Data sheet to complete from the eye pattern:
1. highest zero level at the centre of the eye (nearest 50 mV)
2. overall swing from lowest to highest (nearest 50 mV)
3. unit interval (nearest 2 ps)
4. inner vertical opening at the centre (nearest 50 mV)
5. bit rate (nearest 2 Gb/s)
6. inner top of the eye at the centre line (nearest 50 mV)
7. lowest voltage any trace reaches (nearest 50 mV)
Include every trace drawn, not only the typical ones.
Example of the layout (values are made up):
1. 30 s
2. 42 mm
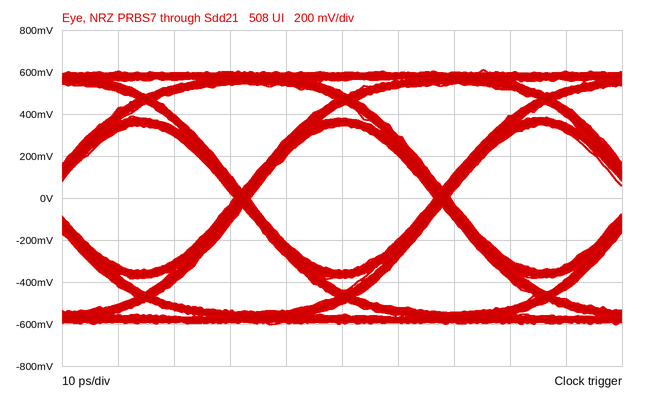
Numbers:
1. -350 mV
2. 1.20 V
3. 36 ps
4. 700 mV
5. 28 Gb/s
6. 350 mV
7. -600 mV
